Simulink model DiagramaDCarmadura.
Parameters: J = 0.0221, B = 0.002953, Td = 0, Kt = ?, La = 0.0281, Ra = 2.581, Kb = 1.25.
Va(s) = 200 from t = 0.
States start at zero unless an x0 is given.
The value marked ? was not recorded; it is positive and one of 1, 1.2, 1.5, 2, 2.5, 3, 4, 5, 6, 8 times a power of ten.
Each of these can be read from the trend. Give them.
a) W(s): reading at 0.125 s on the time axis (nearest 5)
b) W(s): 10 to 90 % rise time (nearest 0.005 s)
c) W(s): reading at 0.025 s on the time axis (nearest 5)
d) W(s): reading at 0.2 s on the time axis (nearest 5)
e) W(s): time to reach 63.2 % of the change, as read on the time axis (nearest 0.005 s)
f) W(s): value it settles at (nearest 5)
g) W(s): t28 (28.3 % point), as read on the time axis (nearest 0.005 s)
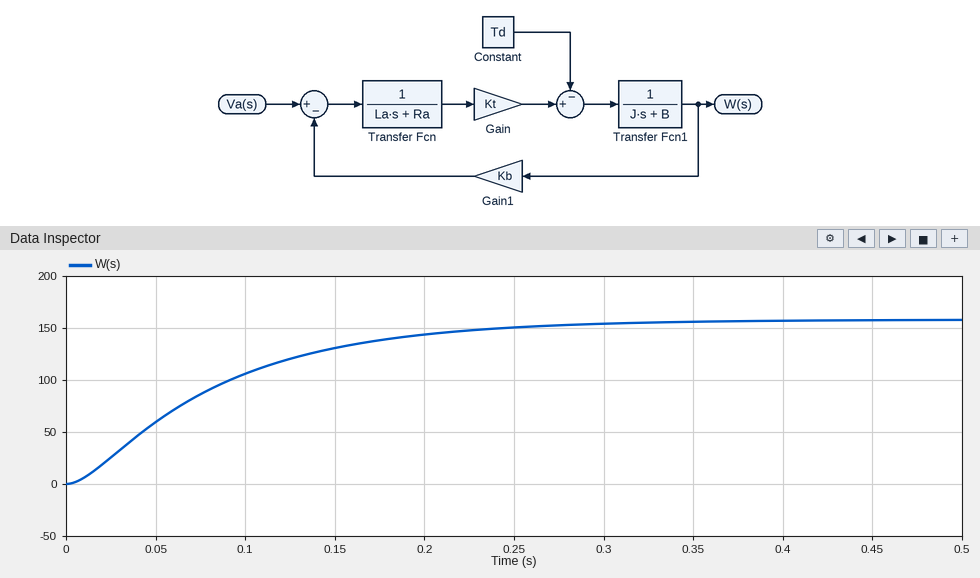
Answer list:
120
0.175 s
25
145
0.090 s
160
0.040 s
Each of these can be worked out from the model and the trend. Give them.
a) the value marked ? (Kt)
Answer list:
0.5
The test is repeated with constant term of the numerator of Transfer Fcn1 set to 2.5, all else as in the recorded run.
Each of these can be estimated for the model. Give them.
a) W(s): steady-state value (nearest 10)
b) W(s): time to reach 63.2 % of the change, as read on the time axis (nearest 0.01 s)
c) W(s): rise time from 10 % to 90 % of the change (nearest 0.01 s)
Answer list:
160
0.04 s
0.06 s
